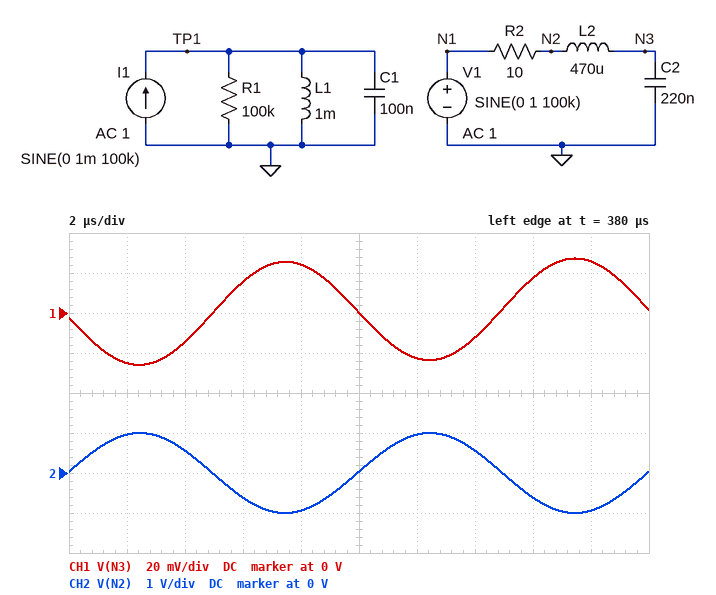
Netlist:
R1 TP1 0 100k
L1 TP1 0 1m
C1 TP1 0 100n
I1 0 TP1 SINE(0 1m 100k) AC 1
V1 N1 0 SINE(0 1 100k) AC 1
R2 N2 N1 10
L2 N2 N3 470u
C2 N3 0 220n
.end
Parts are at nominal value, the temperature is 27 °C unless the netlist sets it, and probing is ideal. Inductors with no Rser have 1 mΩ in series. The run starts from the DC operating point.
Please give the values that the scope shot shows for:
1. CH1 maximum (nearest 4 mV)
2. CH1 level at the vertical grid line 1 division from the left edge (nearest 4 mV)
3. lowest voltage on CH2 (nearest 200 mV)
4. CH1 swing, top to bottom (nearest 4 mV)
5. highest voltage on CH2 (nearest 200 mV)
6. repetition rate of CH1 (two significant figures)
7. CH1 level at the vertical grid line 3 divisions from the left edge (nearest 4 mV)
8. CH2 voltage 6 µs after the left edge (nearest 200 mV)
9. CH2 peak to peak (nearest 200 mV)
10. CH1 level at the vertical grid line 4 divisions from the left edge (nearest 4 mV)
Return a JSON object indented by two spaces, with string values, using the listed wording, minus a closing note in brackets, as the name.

{
  "CH1 maximum": "28 mV",
  "CH1 level at the vertical grid line 1 division from the left edge": "-24 mV",
  "lowest voltage on CH2": "-1.0 V",
  "CH1 swing, top to bottom": "52 mV",
  "highest voltage on CH2": "1.0 V",
  "repetition rate of CH1": "100 kHz",
  "CH1 level at the vertical grid line 3 divisions from the left edge": "16 mV",
  "CH2 voltage 6 µs after the left edge": "-600 mV",
  "CH2 peak to peak": "2.0 V",
  "CH1 level at the vertical grid line 4 divisions from the left edge": "24 mV"
}
